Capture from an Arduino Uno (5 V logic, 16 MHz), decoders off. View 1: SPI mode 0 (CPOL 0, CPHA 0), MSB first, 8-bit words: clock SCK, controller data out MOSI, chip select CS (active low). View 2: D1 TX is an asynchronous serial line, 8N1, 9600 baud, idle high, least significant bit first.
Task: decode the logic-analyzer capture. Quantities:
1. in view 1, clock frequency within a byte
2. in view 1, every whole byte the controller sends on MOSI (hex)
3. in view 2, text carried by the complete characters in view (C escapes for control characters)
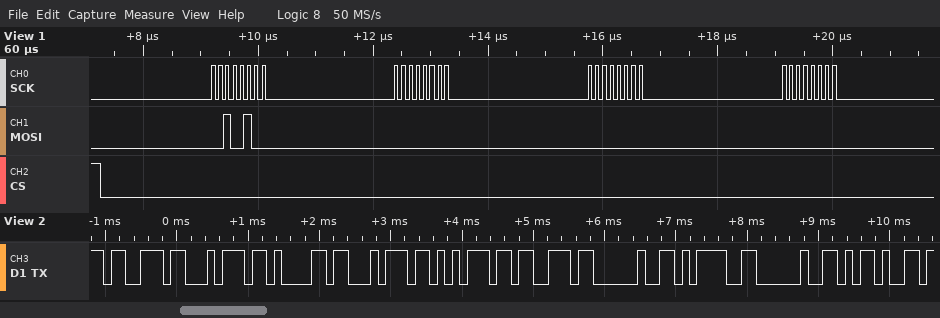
8 MHz
24 00 00 00
"status = -"
